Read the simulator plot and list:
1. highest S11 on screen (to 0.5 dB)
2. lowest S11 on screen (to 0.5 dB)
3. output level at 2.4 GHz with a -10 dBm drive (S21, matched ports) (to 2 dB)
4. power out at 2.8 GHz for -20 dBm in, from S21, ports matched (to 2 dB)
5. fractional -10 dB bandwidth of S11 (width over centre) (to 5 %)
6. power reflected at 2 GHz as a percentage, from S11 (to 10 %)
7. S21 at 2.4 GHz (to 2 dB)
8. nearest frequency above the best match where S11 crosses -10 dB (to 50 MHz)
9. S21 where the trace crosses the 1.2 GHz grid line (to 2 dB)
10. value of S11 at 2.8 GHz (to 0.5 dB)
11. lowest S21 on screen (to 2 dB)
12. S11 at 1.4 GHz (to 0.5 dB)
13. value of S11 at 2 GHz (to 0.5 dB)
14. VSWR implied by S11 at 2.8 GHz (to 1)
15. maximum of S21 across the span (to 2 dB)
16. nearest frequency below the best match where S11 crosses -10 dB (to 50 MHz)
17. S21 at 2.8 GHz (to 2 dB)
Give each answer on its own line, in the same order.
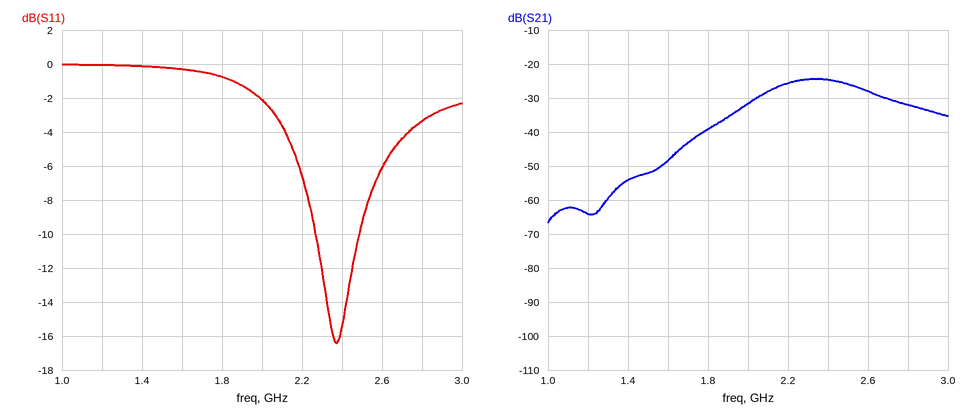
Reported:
0.0 dB
-16.5 dB
-34 dBm
-52 dBm
10 %
60 %
-24 dB
2.50 GHz
-64 dB
-3.5 dB
-66 dB
0.0 dB
-2.0 dB
5
-24 dB
2.25 GHz
-32 dB
